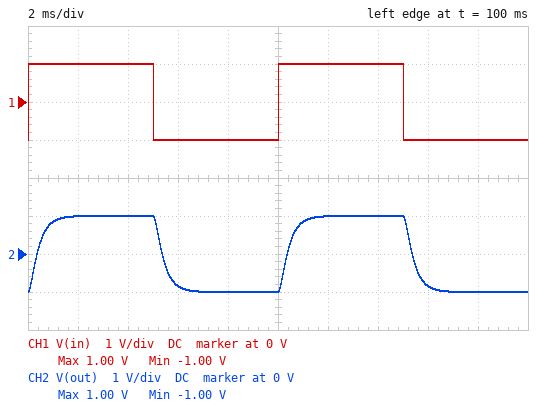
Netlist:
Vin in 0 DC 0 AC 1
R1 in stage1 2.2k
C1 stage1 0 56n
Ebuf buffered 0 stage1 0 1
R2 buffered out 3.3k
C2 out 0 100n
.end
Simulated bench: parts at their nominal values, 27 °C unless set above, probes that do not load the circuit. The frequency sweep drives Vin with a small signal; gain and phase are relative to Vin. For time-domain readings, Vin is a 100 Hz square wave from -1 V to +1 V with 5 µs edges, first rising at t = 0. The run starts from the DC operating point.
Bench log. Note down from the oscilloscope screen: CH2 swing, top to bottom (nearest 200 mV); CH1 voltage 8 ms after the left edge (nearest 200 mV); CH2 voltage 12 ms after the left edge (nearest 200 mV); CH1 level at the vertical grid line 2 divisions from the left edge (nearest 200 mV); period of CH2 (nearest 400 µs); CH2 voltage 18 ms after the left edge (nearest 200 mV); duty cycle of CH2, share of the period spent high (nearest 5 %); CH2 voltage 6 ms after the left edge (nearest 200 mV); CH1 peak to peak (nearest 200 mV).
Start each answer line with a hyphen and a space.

- 2.0 V
- -1.0 V
- 1.0 V
- 1.0 V
- 10.0 ms
- -1.0 V
- 50 %
- -800 mV
- 2.0 V
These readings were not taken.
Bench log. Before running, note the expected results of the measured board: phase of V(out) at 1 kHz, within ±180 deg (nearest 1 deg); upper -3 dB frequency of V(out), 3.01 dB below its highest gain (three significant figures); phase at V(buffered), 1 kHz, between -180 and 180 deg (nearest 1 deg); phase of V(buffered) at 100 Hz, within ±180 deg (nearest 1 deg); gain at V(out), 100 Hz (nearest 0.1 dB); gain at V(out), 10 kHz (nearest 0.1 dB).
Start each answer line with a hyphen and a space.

- -102 deg
- 431 Hz
- -38 deg
- -4 deg
- -0.2 dB
- -44.2 dB
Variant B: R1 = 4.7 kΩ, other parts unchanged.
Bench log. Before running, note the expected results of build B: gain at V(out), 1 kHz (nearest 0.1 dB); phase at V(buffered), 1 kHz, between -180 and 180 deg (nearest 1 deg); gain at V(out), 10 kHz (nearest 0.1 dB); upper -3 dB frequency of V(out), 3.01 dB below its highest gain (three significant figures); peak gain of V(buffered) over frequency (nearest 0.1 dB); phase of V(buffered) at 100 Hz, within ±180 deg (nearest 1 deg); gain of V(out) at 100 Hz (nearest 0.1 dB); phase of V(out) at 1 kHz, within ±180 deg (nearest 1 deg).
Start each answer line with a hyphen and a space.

- -13.0 dB
- -59 deg
- -50.7 dB
- 344 Hz
- 0 dB
- -9 deg
- -0.3 dB
- -123 deg
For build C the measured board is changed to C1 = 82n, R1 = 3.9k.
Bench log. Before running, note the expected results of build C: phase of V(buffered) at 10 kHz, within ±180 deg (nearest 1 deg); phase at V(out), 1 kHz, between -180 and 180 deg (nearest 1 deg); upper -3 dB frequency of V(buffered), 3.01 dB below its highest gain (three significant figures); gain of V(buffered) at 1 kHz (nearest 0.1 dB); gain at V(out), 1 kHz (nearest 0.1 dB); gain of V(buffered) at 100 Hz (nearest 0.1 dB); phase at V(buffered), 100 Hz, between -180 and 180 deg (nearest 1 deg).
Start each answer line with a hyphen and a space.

- -87 deg
- -128 deg
- 498 Hz
- -7.0 dB
- -14.3 dB
- -0.2 dB
- -11 deg
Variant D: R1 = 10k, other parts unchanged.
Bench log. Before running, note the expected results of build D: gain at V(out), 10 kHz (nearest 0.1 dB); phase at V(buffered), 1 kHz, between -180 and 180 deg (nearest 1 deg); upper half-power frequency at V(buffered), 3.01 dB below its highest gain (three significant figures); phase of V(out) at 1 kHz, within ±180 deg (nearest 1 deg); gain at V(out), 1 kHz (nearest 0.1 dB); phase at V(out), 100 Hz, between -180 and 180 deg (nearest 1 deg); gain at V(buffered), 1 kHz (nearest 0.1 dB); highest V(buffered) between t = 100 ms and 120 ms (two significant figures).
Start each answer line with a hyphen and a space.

- -57.3 dB
- -74 deg
- 284 Hz
- -138 deg
- -18.5 dB
- -31 deg
- -11.3 dB
- 1.0 V
